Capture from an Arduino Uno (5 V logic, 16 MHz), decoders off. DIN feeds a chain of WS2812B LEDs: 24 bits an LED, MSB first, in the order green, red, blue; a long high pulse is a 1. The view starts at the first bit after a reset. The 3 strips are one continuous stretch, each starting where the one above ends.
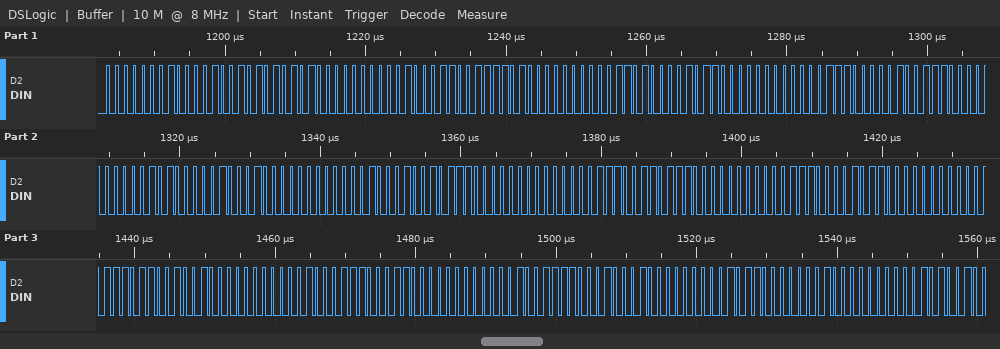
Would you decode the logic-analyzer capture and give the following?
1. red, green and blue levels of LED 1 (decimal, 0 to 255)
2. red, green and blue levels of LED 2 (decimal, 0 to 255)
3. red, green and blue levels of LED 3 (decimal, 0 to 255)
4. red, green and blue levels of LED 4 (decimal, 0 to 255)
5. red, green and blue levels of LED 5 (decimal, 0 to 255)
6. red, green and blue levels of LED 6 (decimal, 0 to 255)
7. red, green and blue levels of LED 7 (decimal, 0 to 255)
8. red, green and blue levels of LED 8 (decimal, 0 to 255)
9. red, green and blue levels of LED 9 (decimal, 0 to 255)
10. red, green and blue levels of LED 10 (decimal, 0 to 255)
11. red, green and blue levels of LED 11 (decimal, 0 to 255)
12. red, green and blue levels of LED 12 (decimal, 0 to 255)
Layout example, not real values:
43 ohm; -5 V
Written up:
9, 1, 85; 35, 0, 61; 52, 0, 44; 56, 0, 39; 40, 0, 34; 17, 0, 46; 7, 0, 55; 28, 0, 44; 59, 0, 36; 71, 0, 24; 79, 0, 17; 88, 0, 8
